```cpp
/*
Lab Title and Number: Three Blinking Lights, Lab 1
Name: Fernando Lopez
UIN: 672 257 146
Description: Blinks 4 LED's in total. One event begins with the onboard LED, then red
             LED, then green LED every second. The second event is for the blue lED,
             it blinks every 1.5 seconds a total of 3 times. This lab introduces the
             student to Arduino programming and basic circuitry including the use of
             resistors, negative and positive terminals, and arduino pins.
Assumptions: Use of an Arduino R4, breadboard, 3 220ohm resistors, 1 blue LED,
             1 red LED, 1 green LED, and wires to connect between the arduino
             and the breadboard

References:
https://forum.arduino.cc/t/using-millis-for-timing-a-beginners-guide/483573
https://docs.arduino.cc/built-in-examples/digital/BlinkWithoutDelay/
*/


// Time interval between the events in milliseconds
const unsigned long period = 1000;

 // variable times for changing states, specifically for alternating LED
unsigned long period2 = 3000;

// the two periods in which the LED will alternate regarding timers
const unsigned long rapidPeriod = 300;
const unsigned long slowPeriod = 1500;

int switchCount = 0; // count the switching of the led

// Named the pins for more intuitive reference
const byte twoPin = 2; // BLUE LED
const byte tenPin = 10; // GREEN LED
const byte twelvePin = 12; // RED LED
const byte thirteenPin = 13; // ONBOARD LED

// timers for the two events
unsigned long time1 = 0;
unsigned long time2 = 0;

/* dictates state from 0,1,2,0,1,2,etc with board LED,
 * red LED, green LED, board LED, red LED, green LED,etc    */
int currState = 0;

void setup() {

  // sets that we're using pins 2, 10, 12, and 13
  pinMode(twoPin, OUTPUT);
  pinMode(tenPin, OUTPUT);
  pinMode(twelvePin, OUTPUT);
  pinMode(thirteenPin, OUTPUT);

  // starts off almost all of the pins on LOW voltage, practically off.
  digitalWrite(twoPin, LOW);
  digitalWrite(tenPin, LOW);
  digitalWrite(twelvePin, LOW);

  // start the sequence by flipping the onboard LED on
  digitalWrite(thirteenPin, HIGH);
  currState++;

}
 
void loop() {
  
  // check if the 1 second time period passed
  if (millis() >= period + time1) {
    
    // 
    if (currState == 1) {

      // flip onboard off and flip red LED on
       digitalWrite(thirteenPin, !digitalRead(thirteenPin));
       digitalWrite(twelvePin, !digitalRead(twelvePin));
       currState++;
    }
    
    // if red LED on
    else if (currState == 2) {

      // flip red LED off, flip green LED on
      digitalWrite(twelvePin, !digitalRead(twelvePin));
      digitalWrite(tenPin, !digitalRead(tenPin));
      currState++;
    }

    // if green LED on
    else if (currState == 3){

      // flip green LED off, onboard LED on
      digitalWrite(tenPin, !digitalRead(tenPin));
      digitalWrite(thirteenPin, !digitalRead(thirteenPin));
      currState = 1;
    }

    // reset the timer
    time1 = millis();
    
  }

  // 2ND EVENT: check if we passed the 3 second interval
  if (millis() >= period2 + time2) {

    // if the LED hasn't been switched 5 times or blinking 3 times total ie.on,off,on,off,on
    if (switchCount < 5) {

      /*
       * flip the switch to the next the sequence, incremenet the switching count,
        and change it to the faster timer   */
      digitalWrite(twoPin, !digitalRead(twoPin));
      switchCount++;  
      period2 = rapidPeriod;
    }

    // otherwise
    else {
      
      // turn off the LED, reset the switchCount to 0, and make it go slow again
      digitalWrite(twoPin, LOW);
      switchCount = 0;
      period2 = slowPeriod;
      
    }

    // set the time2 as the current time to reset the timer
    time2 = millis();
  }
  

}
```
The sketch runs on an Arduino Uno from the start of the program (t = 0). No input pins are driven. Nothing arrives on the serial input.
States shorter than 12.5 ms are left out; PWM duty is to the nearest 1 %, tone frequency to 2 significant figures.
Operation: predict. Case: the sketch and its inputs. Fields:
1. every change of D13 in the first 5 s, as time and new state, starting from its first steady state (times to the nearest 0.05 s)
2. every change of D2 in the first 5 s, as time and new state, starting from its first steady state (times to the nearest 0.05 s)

0 s high; 1 s low; 3 s high; 4 s low
0 s low; 3 s high; 3.3 s low; 3.6 s high; 3.9 s low; 4.2 s high; 4.5 s low
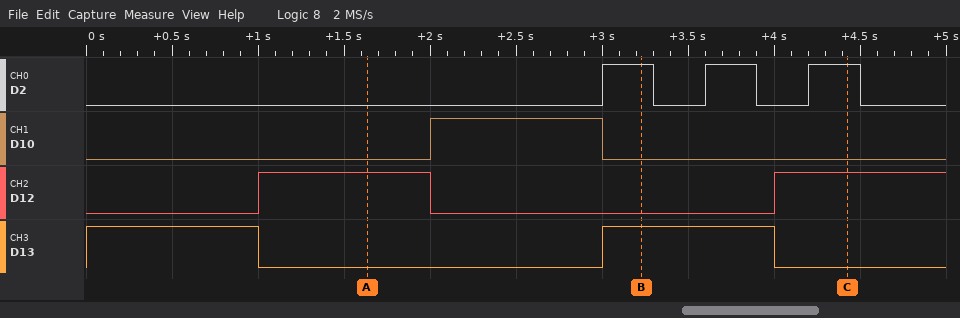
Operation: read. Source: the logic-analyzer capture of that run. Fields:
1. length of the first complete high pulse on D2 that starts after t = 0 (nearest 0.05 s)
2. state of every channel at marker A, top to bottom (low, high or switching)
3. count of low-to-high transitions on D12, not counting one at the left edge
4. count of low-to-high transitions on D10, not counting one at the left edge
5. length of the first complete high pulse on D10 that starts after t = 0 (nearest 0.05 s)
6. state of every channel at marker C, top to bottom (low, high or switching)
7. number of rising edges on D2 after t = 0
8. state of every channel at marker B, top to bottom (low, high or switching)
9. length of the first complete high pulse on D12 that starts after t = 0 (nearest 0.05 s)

0.30 s
D2 low, D10 low, D12 high, D13 low
2
1
1.00 s
D2 high, D10 low, D12 high, D13 low
3
D2 high, D10 low, D12 low, D13 high
1.00 s
